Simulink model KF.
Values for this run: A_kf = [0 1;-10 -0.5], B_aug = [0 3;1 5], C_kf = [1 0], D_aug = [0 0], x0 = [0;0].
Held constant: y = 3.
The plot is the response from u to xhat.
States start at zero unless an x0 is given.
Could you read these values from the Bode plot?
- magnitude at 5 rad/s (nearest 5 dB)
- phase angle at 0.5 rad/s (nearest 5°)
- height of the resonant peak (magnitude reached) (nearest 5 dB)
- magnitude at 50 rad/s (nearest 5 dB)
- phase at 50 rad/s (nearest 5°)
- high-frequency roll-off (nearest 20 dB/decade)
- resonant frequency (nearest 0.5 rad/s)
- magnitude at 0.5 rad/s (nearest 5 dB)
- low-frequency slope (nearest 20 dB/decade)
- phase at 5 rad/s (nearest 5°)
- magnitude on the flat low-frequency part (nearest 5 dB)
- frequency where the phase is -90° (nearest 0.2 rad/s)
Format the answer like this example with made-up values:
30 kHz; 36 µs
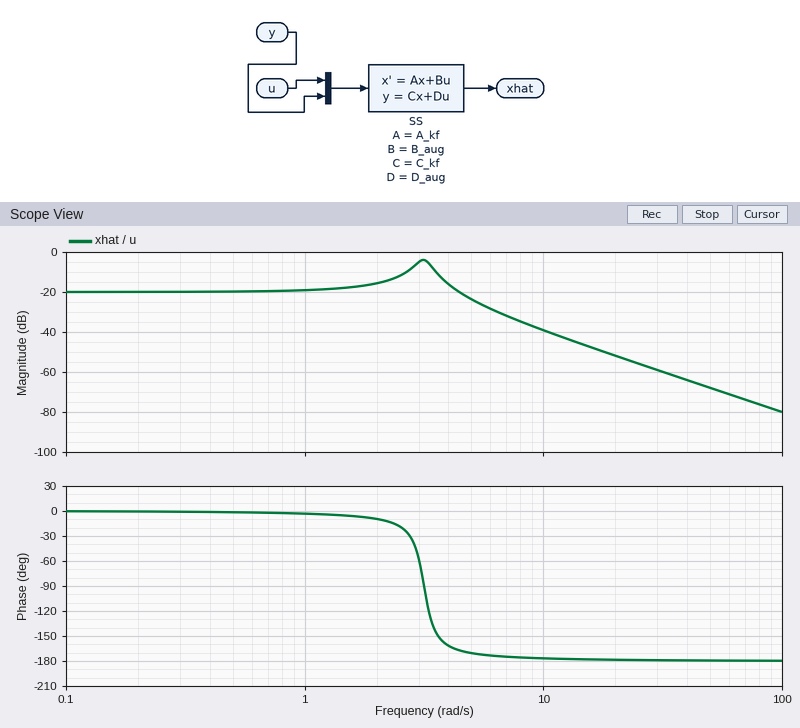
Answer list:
-25 dB; 0°; -5 dB; -70 dB; -180°; -40 dB/decade; 3.0 rad/s; -20 dB; 0 dB/decade; -170°; -20 dB; 3.2 rad/s
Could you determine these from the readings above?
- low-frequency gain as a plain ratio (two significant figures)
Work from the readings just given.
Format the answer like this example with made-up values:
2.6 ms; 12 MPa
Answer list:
0.10
